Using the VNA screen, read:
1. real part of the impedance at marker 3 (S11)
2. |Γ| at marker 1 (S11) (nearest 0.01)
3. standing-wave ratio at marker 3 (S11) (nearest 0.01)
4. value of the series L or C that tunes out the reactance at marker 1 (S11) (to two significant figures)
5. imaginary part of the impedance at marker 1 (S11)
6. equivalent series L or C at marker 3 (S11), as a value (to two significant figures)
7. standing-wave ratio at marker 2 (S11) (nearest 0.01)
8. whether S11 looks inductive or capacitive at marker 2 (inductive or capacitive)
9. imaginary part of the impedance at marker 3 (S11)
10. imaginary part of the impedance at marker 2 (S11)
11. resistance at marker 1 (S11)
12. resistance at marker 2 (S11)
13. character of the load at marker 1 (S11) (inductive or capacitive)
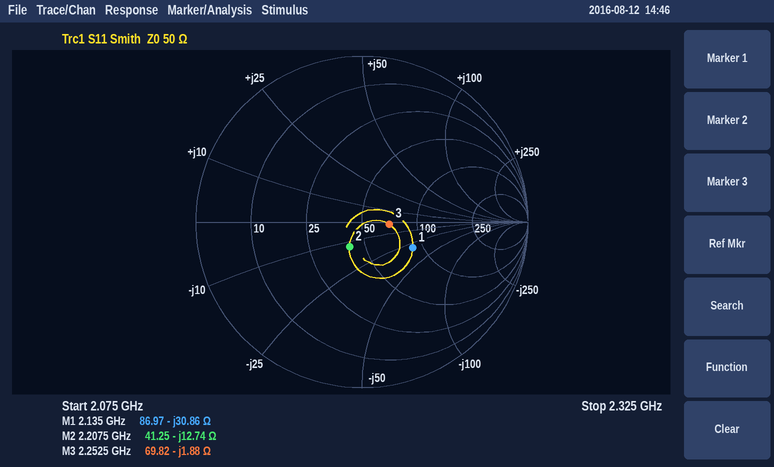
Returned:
69.82 Ω
0.34
1.40
2.3 nH
-30.86 Ω
38 pF
1.40
capacitive
-1.88 Ω
-12.74 Ω
86.97 Ω
41.25 Ω
capacitive
